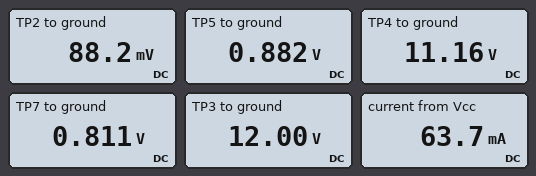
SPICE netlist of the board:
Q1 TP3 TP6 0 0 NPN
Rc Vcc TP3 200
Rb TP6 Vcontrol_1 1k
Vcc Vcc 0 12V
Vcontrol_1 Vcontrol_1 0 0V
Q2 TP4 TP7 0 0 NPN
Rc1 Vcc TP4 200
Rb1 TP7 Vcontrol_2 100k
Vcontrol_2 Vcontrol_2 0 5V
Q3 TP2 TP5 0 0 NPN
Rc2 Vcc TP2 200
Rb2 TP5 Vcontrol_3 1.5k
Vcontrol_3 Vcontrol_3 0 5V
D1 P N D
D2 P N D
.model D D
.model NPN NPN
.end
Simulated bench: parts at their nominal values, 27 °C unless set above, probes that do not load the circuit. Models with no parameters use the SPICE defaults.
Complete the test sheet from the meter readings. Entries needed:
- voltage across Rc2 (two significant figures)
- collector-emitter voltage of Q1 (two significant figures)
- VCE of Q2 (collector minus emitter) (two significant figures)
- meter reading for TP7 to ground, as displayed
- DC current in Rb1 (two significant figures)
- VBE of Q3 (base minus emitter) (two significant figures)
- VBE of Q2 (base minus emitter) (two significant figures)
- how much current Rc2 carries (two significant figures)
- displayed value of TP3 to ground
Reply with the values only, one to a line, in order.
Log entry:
12 V
12 V
11 V
0.811 V
42 µA
880 mV
810 mV
60 mA
12.00 V
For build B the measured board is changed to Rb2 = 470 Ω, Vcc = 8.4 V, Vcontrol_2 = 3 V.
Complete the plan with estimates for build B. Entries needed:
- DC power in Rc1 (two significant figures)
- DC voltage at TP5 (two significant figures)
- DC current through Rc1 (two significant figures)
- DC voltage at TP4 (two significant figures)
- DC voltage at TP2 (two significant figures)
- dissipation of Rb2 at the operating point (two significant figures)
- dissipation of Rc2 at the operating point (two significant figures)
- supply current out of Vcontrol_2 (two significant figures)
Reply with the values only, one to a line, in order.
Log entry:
970 µW
880 mV
2.2 mA
8.0 V
51 mV
36 mW
350 mW
22 µA
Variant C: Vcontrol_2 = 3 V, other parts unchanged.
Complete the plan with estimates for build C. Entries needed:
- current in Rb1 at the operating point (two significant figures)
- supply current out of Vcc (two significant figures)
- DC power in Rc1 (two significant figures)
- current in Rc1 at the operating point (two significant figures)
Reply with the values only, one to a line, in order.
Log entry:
22 µA
62 mA
970 µW
2.2 mA
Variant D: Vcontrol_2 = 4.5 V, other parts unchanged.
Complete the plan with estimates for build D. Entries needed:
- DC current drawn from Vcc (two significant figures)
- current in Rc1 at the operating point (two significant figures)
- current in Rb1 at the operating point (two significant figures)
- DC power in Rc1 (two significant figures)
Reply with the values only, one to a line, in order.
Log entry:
63 mA
3.7 mA
37 µA
2.7 mW
